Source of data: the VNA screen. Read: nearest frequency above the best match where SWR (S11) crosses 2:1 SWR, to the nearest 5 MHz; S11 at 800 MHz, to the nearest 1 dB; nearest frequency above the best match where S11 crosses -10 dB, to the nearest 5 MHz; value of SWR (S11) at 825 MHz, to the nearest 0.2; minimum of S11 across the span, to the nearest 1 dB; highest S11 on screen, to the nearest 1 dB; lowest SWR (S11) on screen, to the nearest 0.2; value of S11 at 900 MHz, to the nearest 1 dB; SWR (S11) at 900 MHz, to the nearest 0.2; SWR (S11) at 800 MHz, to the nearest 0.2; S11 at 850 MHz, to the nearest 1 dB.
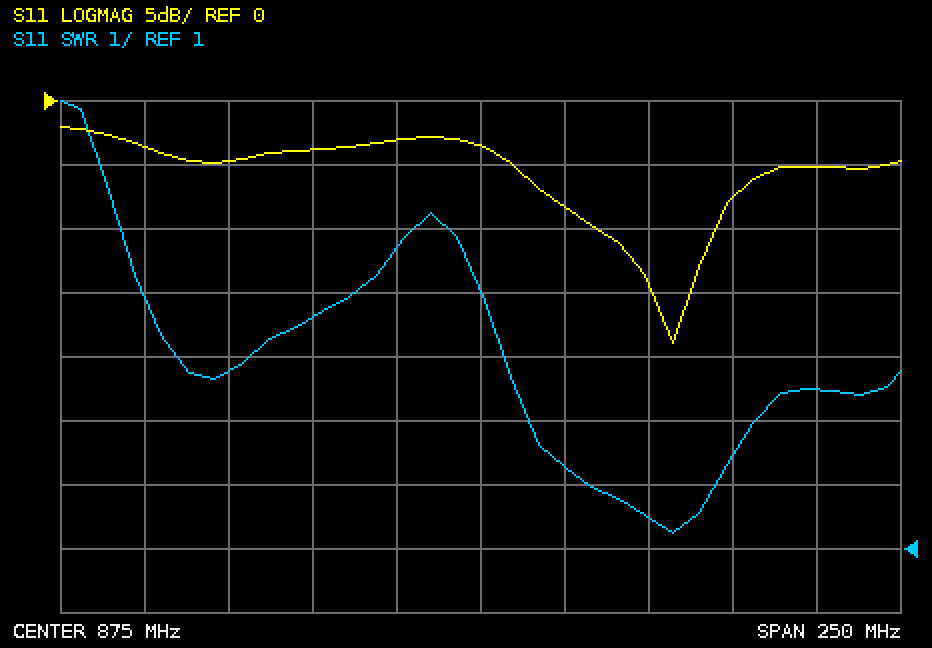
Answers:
945 MHz
-5 dB
945 MHz
4.6
-19 dB
-2 dB
1.2
-8 dB
2.2
3.8
-3 dB
